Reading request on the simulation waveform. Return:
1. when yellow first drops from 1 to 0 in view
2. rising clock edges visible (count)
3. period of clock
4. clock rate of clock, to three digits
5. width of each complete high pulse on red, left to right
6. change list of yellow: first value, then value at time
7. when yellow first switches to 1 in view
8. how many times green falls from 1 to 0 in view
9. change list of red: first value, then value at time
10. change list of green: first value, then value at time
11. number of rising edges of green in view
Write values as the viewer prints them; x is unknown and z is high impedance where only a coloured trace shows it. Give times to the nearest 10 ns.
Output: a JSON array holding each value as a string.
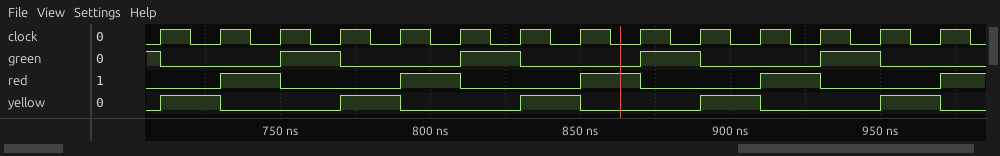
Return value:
["730 ns", "14", "20 ns", "50.0 MHz", "20 ns, 20 ns, 20 ns, 20 ns", "0, 1 at 710 ns, 0 at 730 ns, 1 at 770 ns, 0 at 790 ns, 1 at 830 ns, 0 at 850 ns, 1 at 890 ns, 0 at 910 ns, 1 at 950 ns, 0 at 970 ns", "710 ns", "5", "0, 1 at 730 ns, 0 at 750 ns, 1 at 790 ns, 0 at 810 ns, 1 at 850 ns, 0 at 870 ns, 1 at 910 ns, 0 at 930 ns, 1 at 970 ns", "1, 0 at 710 ns, 1 at 750 ns, 0 at 770 ns, 1 at 810 ns, 0 at 830 ns, 1 at 870 ns, 0 at 890 ns, 1 at 930 ns, 0 at 950 ns", "4"]
